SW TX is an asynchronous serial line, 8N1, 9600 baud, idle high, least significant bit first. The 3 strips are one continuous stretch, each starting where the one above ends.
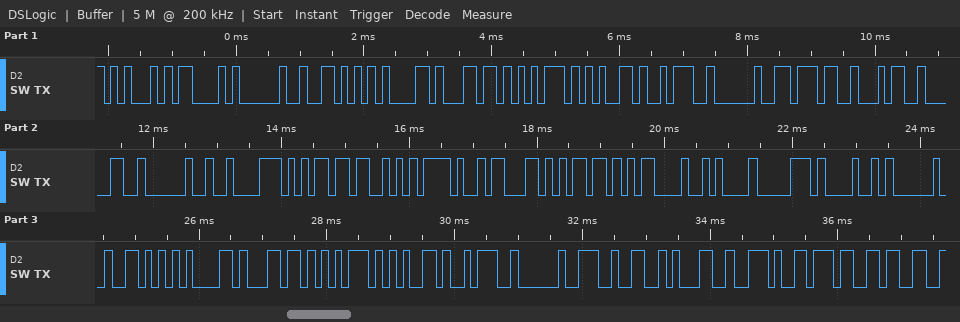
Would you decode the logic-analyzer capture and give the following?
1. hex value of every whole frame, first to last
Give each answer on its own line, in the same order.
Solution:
45 43 20 56 61 6C 75 65 3A 20 37 34 30 20 C2 B5 53 2F 63 6D 0D 0A 70 48 20 56 61 6C 75 65 3A 20 32 31 2E 37 33
